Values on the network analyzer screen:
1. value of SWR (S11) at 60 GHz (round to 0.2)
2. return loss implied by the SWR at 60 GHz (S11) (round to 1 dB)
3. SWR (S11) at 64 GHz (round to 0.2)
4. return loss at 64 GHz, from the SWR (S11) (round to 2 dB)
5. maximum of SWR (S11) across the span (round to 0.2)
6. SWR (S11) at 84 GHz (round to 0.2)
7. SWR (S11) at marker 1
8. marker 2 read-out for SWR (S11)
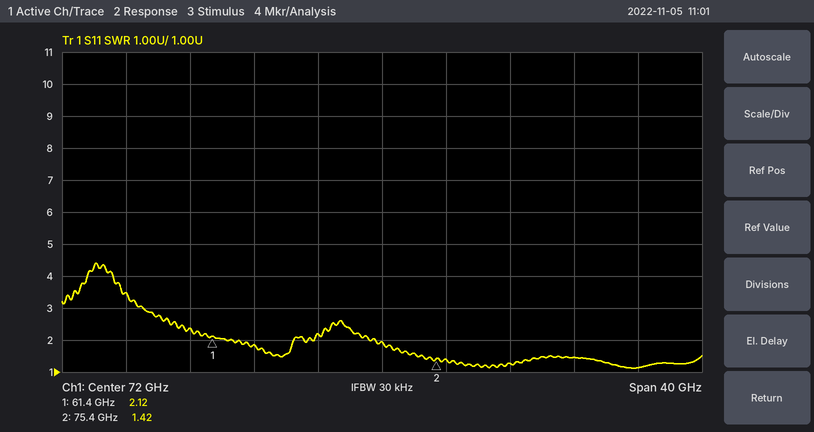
2.4
8 dB
1.8
10 dB
4.4
1.4
2.12
1.42
